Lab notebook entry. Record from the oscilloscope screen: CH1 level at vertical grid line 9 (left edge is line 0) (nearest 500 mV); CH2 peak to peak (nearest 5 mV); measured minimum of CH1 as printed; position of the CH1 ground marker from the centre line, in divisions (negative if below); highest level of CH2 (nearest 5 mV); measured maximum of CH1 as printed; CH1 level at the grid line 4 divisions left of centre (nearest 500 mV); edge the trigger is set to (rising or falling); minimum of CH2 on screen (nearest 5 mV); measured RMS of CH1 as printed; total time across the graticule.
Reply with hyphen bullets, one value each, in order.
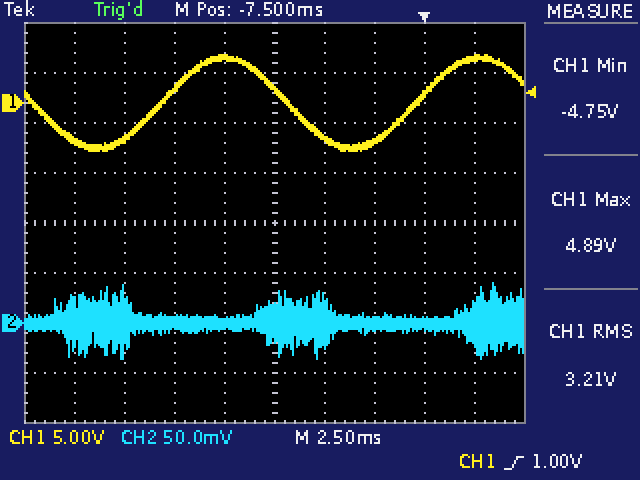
- 4.5 V
- 75 mV
- -4.75 V
- +2.4 div
- 40 mV
- 4.89 V
- -3.5 V
- rising
- -35 mV
- 3.21 V
- 25 ms
